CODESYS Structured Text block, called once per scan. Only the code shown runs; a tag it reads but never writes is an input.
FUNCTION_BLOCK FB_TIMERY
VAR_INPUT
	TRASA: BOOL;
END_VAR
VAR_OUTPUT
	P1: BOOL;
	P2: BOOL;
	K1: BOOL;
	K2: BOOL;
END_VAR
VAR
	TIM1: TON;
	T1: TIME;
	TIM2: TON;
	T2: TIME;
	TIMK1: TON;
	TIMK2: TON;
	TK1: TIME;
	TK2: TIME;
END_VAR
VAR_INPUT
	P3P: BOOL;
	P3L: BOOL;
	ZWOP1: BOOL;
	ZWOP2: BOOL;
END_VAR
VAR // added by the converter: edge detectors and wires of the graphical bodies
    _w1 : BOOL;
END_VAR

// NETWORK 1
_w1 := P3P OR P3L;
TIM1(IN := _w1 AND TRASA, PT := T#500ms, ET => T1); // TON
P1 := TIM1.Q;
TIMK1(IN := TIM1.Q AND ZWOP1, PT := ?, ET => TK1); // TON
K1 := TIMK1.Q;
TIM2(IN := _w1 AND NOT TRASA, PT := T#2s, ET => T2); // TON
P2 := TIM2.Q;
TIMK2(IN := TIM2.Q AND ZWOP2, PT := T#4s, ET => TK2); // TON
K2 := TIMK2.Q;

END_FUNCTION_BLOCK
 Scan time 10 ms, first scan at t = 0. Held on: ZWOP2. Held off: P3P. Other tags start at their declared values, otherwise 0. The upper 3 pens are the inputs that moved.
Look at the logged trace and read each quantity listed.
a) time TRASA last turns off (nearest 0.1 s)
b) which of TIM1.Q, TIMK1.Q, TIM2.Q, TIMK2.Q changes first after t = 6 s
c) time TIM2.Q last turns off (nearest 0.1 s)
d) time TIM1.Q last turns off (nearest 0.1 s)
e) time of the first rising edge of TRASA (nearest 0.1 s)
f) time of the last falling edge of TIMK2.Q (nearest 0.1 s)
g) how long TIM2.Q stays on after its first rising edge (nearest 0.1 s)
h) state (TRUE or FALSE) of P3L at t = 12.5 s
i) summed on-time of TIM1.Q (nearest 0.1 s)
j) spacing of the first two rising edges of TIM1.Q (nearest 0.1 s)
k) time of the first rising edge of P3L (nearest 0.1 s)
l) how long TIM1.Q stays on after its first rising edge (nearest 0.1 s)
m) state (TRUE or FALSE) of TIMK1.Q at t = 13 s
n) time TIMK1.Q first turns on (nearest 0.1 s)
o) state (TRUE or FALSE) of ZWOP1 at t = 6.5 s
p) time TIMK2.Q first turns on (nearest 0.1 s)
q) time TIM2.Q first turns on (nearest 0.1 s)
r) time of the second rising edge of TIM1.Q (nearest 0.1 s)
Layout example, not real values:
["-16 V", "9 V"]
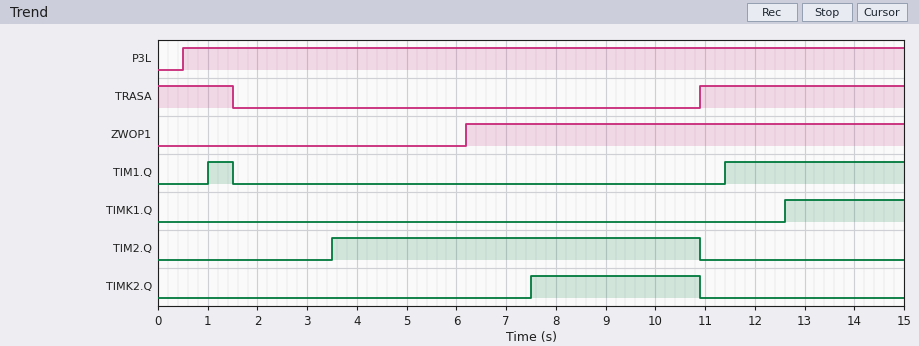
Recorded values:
["1.5 s", "TIMK2.Q", "10.9 s", "1.5 s", "10.9 s", "10.9 s", "7.4 s", "TRUE", "4.1 s", "10.4 s", "0.5 s", "0.5 s", "TRUE", "12.6 s", "TRUE", "7.5 s", "3.5 s", "11.4 s"]
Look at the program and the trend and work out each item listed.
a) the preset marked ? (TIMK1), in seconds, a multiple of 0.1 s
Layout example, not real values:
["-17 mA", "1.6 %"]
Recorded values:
["1.2 s"]
